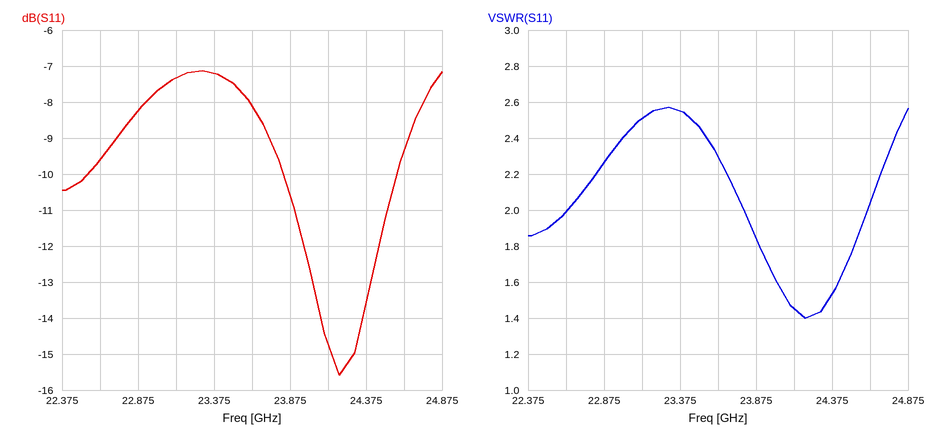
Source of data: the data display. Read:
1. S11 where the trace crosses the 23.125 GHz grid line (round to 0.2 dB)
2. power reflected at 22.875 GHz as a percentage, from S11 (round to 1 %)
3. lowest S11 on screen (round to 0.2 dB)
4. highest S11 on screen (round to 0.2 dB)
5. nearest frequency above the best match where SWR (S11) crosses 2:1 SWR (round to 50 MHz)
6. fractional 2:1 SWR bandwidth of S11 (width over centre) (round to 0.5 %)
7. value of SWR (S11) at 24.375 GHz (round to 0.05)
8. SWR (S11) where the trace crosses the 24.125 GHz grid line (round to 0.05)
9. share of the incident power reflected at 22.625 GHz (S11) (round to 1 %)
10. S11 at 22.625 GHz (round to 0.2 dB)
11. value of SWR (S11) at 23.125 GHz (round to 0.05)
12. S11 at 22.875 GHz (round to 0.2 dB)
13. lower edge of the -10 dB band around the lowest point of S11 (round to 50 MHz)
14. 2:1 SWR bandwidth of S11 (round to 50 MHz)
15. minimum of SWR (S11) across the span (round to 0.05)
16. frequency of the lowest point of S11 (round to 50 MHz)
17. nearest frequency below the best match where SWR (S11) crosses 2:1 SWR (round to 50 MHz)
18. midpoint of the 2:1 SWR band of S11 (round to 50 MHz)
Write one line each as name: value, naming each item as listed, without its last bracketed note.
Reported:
S11 where the trace crosses the 23.125 GHz grid line: -7.4 dB
power reflected at 22.875 GHz as a percentage, from S11: 15 %
lowest S11 on screen: -15.6 dB
highest S11 on screen: -7.2 dB
nearest frequency above the best match where SWR (S11) crosses 2:1 SWR: 24.60 GHz
fractional 2:1 SWR bandwidth of S11 (width over centre): 3.5 %
value of SWR (S11) at 24.375 GHz: 1.55
SWR (S11) where the trace crosses the 24.125 GHz grid line: 1.45
share of the incident power reflected at 22.625 GHz (S11): 11 %
S11 at 22.625 GHz: -9.6 dB
value of SWR (S11) at 23.125 GHz: 2.50
S11 at 22.875 GHz: -8.2 dB
lower edge of the -10 dB band around the lowest point of S11: 23.85 GHz
2:1 SWR bandwidth of S11: 800 MHz
minimum of SWR (S11) across the span: 1.40
frequency of the lowest point of S11: 24.20 GHz
nearest frequency below the best match where SWR (S11) crosses 2:1 SWR: 23.80 GHz
midpoint of the 2:1 SWR band of S11: 24.20 GHz
